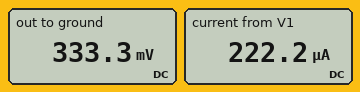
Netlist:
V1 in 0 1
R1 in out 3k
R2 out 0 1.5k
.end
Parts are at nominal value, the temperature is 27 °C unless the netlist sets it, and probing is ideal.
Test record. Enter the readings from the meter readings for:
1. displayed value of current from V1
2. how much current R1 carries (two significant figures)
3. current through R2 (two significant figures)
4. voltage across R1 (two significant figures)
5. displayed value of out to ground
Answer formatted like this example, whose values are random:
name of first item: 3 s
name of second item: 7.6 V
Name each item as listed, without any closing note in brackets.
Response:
displayed value of current from V1: 222.2 µA
how much current R1 carries: 220 µA
current through R2: 220 µA
voltage across R1: 670 mV
displayed value of out to ground: 333.3 mV
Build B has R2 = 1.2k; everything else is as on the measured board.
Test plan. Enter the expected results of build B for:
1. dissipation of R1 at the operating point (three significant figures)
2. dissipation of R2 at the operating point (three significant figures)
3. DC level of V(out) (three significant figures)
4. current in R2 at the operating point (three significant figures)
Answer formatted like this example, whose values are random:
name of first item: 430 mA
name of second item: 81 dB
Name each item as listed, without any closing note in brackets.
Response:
dissipation of R1 at the operating point: 170 µW
dissipation of R2 at the operating point: 68.0 µW
DC level of V(out): 286 mV
current in R2 at the operating point: 238 µA
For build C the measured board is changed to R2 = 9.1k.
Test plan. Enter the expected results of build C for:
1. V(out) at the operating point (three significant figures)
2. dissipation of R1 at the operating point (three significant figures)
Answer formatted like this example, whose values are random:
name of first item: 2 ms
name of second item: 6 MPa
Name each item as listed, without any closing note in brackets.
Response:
V(out) at the operating point: 752 mV
dissipation of R1 at the operating point: 20.5 µW
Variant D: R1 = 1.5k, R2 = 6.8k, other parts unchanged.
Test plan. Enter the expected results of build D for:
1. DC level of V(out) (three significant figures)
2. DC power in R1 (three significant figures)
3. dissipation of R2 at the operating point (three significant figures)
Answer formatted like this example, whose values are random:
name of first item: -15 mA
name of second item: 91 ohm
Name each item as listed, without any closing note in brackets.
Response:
DC level of V(out): 819 mV
DC power in R1: 21.8 µW
dissipation of R2 at the operating point: 98.7 µW
